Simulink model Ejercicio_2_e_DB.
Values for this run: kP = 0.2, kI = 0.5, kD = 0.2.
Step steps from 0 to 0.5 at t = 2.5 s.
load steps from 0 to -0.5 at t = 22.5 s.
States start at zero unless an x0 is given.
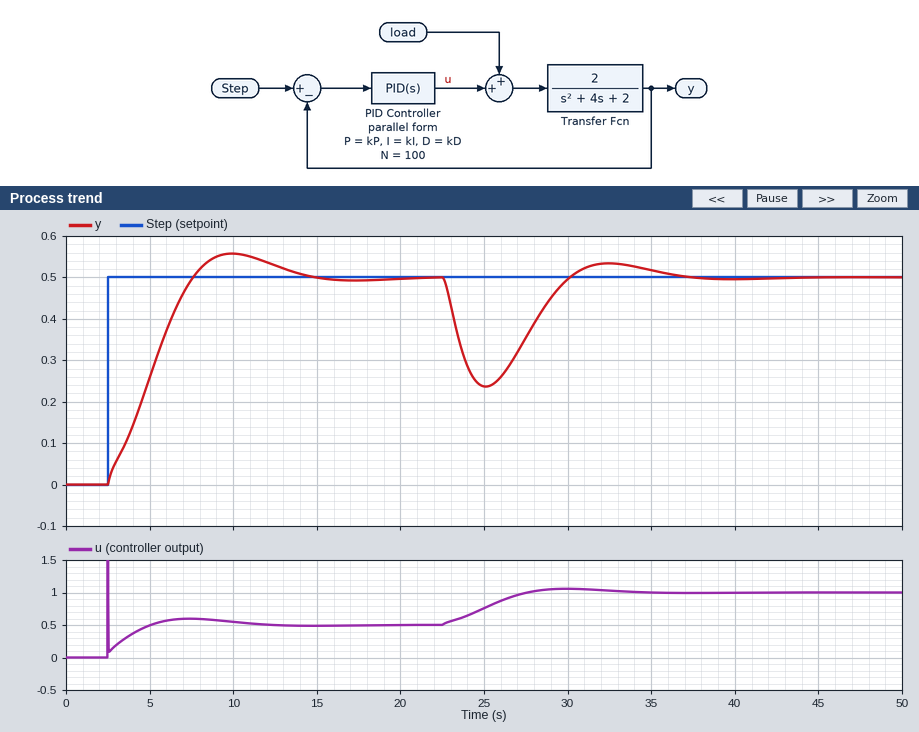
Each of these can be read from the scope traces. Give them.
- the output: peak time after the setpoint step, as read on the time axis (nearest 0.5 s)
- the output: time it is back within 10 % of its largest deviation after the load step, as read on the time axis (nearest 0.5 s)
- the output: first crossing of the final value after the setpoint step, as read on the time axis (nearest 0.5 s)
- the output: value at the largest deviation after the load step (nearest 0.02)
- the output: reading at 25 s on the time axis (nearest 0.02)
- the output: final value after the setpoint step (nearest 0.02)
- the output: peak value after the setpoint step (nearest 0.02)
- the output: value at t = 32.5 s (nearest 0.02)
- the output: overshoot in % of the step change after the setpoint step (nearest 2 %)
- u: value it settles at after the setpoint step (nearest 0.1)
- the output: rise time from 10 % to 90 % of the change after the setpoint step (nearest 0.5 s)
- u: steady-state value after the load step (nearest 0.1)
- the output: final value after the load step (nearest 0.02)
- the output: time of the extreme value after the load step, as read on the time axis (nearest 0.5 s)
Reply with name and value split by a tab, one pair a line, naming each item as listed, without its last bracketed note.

the output: peak time after the setpoint step, as read on the time axis	10.0 s
the output: time it is back within 10 % of its largest deviation after the load step, as read on the time axis	34.0 s
the output: first crossing of the final value after the setpoint step, as read on the time axis	7.5 s
the output: value at the largest deviation after the load step	0.24
the output: reading at 25 s on the time axis	0.24
the output: final value after the setpoint step	0.50
the output: peak value after the setpoint step	0.56
the output: value at t = 32.5 s	0.54
the output: overshoot in % of the step change after the setpoint step	12 %
u: value it settles at after the setpoint step	0.5
the output: rise time from 10 % to 90 % of the change after the setpoint step	4.0 s
u: steady-state value after the load step	1.0
the output: final value after the load step	0.50
the output: time of the extreme value after the load step, as read on the time axis	25.0 s
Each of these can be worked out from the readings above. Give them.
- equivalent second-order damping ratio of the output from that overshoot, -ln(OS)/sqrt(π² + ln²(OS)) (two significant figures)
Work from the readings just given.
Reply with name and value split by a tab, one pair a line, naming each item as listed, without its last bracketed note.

equivalent second-order damping ratio of the output from that overshoot, -ln(OS)/sqrt(π² + ln²(OS))	0.56
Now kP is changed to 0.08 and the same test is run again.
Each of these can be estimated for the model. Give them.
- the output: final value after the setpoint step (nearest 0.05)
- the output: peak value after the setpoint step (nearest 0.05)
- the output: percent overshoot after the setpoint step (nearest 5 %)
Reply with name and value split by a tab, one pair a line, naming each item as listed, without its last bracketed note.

the output: final value after the setpoint step	0.50
the output: peak value after the setpoint step	0.60
the output: percent overshoot after the setpoint step	15 %
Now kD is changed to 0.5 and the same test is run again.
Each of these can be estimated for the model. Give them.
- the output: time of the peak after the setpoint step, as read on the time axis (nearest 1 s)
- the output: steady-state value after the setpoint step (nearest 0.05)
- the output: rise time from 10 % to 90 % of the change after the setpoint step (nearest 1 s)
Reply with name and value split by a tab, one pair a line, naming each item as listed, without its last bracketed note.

the output: time of the peak after the setpoint step, as read on the time axis	11 s
the output: steady-state value after the setpoint step	0.50
the output: rise time from 10 % to 90 % of the change after the setpoint step	5 s
